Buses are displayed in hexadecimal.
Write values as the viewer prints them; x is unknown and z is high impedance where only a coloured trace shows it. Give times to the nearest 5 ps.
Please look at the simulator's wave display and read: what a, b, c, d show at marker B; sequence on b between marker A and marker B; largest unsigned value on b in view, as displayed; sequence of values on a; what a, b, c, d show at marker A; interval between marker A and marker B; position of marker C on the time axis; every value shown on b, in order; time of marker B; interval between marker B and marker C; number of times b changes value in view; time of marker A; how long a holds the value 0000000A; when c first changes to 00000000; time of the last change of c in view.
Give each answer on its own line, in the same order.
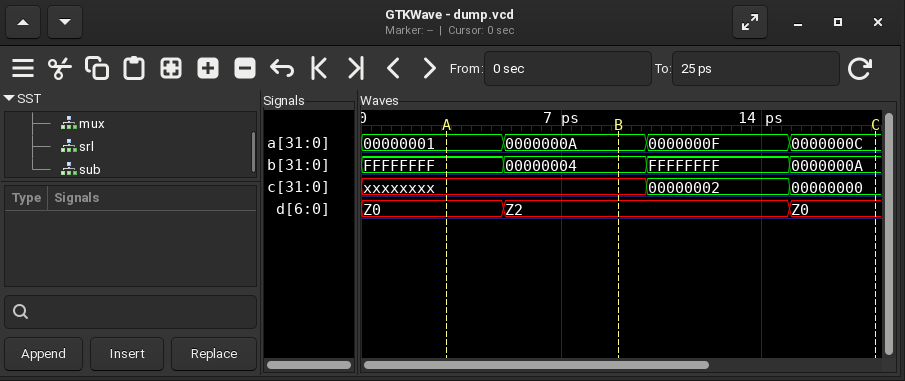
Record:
a=0000000A, b=00000004, c=xxxxxxxx, d=Z2
FFFFFFFF, 00000004
FFFFFFFF
00000001, 0000000A, 0000000F, 0000000C
a=00000001, b=FFFFFFFF, c=xxxxxxxx, d=Z0
5 ps
20 ps
FFFFFFFF, 00000004, FFFFFFFF, 0000000A
10 ps
10 ps
3
5 ps
5 ps
15 ps
15 ps
